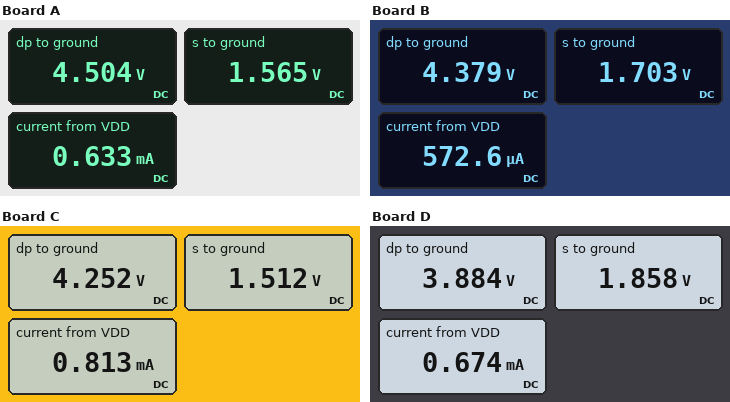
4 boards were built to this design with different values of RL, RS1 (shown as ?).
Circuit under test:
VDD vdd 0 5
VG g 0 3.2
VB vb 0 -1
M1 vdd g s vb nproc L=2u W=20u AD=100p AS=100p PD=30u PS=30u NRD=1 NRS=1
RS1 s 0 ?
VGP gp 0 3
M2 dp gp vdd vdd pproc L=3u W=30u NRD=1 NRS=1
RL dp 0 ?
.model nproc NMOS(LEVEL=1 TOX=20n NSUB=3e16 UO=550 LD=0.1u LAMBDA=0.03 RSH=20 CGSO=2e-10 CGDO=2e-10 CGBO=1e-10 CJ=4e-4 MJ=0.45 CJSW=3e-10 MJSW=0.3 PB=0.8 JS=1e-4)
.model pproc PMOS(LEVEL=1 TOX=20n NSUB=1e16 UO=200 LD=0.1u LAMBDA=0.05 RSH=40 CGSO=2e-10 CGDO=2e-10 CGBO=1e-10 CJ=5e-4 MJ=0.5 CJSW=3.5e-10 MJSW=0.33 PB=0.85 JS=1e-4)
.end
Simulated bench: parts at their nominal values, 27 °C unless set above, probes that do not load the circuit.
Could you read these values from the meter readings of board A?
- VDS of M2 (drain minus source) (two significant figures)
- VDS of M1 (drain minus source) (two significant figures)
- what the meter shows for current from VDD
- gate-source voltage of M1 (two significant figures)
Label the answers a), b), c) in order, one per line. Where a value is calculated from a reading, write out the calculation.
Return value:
a) 4.504 V - 5 V = -500 mV
b) 5 V - 1.565 V = 3.4 V
c) 0.633 mA
d) 3.2 V - 1.565 V = 1.6 V
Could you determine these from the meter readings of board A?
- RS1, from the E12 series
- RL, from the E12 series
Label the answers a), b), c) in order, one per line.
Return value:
a) 4.7 kΩ
b) 15 kΩ
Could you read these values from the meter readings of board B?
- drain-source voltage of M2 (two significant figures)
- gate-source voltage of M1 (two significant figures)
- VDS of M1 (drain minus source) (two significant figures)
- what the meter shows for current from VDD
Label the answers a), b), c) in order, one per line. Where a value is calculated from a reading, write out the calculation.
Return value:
a) 4.379 V - 5 V = -620 mV
b) 3.2 V - 1.703 V = 1.5 V
c) 5 V - 1.703 V = 3.3 V
d) 572.6 µA
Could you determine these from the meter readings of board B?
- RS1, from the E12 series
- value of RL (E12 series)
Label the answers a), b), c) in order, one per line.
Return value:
a) 8.2 kΩ
b) 12 kΩ
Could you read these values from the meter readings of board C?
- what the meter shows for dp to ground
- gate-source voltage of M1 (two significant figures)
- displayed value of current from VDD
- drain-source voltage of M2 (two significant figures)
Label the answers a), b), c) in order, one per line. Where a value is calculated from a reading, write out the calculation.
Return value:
a) 4.252 V
b) 3.2 V - 1.512 V = 1.7 V
c) 0.813 mA
d) 4.252 V - 5 V = -750 mV
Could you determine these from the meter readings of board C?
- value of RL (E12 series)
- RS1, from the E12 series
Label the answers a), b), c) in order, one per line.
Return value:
a) 10 kΩ
b) 3.9 kΩ
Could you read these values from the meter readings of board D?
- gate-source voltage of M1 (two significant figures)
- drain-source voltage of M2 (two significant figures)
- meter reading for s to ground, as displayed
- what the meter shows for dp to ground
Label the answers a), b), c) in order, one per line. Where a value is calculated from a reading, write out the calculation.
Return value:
a) 3.2 V - 1.858 V = 1.3 V
b) 3.884 V - 5 V = -1.1 V
c) 1.858 V
d) 3.884 V
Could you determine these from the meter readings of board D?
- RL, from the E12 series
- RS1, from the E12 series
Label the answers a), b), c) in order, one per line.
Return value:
a) 6.8 kΩ
b) 18 kΩ
